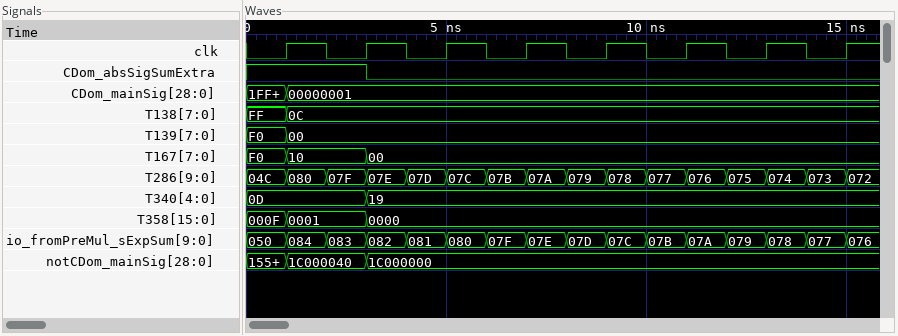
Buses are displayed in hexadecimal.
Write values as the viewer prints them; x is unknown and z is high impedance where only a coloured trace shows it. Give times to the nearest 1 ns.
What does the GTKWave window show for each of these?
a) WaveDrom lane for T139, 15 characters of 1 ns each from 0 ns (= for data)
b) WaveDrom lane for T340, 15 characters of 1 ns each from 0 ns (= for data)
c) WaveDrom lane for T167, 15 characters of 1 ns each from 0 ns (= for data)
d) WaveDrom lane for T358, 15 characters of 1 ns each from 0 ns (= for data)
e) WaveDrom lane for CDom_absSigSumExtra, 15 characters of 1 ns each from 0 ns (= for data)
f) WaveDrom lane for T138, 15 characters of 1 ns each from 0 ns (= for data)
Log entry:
{name: 'T139', wave: '==.............', data: 'F0 00'}
{name: 'T340', wave: '=..=...........', data: '0D 19'}
{name: 'T167', wave: '==.=...........', data: 'F0 10 00'}
{name: 'T358', wave: '==.=...........', data: '000F 0001 0000'}
{name: 'CDom_absSigSumExtra', wave: '1..0...........'}
{name: 'T138', wave: '==.............', data: 'FF 0C'}
